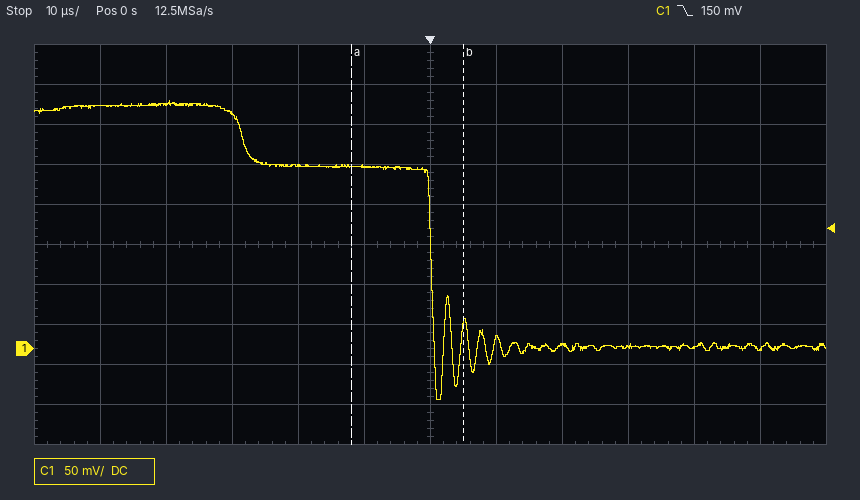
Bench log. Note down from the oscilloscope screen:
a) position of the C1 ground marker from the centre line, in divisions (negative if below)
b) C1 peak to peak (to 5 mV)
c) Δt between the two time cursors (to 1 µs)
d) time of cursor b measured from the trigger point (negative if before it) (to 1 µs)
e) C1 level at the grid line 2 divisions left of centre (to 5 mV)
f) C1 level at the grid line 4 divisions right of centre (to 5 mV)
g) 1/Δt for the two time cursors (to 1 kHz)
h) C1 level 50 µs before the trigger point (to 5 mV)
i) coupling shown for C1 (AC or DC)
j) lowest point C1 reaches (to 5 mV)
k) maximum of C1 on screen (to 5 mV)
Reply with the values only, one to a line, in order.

-2.6 div
375 mV
17 µs
+5 µs
230 mV
0 mV
59 kHz
305 mV
DC
-65 mV
310 mV
